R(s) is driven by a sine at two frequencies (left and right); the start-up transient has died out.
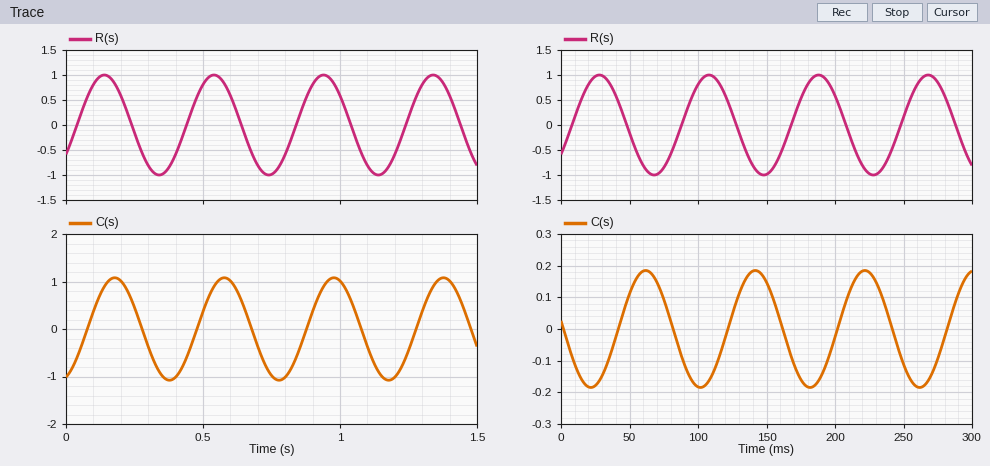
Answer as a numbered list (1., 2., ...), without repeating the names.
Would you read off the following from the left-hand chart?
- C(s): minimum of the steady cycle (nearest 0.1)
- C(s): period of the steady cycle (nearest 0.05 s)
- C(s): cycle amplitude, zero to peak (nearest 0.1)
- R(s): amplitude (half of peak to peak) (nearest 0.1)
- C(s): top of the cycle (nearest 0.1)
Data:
1. -1.1
2. 0.40 s
3. 1.1
4. 1.0
5. 1.1
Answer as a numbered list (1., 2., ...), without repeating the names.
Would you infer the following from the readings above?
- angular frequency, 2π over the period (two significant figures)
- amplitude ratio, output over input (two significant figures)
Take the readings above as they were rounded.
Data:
1. 16 rad/s
2. 1.1
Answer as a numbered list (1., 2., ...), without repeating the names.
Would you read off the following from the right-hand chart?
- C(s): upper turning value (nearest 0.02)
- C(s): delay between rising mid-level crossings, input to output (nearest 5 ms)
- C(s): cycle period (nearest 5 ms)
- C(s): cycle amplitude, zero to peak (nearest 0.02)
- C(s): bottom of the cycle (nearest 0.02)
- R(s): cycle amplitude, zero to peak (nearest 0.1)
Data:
1. 0.18
2. 35 ms
3. 80 ms
4. 0.18
5. -0.18
6. 1.0
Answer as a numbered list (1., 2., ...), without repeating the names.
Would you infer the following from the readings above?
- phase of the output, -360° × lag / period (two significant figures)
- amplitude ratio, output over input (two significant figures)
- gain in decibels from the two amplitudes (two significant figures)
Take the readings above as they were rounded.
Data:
1. -160°
2. 0.18
3. -15 dB
